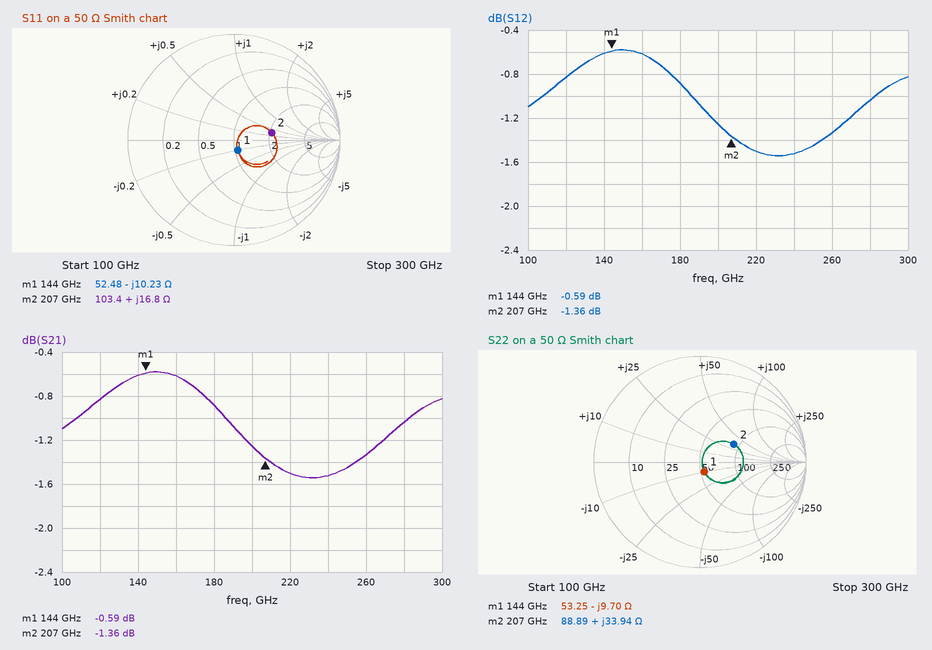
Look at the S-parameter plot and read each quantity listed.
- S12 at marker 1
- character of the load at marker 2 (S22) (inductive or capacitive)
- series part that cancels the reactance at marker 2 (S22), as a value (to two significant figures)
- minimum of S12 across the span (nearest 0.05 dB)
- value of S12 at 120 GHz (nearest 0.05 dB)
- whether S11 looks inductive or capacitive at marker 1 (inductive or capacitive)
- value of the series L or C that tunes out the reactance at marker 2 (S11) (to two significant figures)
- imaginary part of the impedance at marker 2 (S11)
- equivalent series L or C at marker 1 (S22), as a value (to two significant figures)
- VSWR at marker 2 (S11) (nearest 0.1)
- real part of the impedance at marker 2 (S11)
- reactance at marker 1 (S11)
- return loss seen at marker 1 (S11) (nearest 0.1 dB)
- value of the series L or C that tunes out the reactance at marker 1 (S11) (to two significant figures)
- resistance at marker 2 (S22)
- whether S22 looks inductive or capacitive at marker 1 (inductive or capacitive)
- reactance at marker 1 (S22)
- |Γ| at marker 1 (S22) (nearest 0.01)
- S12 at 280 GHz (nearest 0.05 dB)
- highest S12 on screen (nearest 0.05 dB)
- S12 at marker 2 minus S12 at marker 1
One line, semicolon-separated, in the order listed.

-0.59 dB; inductive; 23 fF; -1.55 dB; -0.85 dB; capacitive; 46 fF; +16.8 Ω; 110 fF; 2.1; 103.4 Ω; -10.23 Ω; 19.8 dB; 11 pH; 88.89 Ω; capacitive; -9.70 Ω; 0.10; -1.05 dB; -0.60 dB; -0.77 dB
